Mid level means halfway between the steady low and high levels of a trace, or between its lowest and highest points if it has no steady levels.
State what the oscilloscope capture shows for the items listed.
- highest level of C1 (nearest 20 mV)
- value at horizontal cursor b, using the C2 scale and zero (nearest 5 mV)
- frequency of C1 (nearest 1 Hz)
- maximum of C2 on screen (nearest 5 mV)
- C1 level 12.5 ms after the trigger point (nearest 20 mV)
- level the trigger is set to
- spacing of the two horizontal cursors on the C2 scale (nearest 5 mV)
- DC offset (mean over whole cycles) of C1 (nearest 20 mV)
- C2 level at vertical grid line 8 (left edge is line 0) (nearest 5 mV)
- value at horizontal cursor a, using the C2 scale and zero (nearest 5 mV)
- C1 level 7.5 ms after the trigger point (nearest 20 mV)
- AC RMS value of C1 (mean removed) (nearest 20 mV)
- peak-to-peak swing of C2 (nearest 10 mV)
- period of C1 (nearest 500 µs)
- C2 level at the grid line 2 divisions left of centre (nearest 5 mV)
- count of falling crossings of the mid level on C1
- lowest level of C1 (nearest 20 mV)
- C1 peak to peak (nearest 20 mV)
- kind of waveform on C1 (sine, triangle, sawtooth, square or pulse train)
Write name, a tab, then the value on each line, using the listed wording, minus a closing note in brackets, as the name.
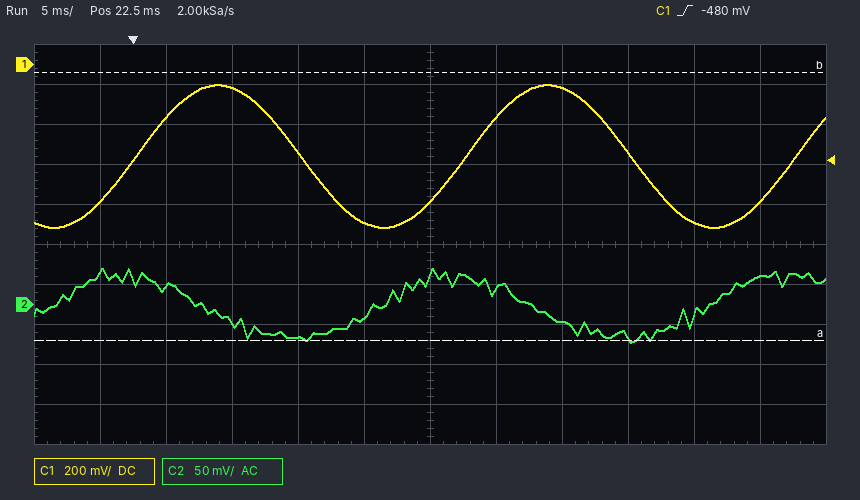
highest level of C1	-100 mV
value at horizontal cursor b, using the C2 scale and zero	290 mV
frequency of C1	40 Hz
maximum of C2 on screen	45 mV
C1 level 12.5 ms after the trigger point	-440 mV
level the trigger is set to	-480 mV
spacing of the two horizontal cursors on the C2 scale	335 mV
DC offset (mean over whole cycles) of C1	-460 mV
C2 level at vertical grid line 8 (left edge is line 0)	-20 mV
value at horizontal cursor a, using the C2 scale and zero	-45 mV
C1 level 7.5 ms after the trigger point	-120 mV
AC RMS value of C1 (mean removed)	260 mV
peak-to-peak swing of C2	90 mV
period of C1	25.0 ms
C2 level at the grid line 2 divisions left of centre	-40 mV
count of falling crossings of the mid level on C1	2
lowest level of C1	-820 mV
C1 peak to peak	720 mV
kind of waveform on C1	sine
